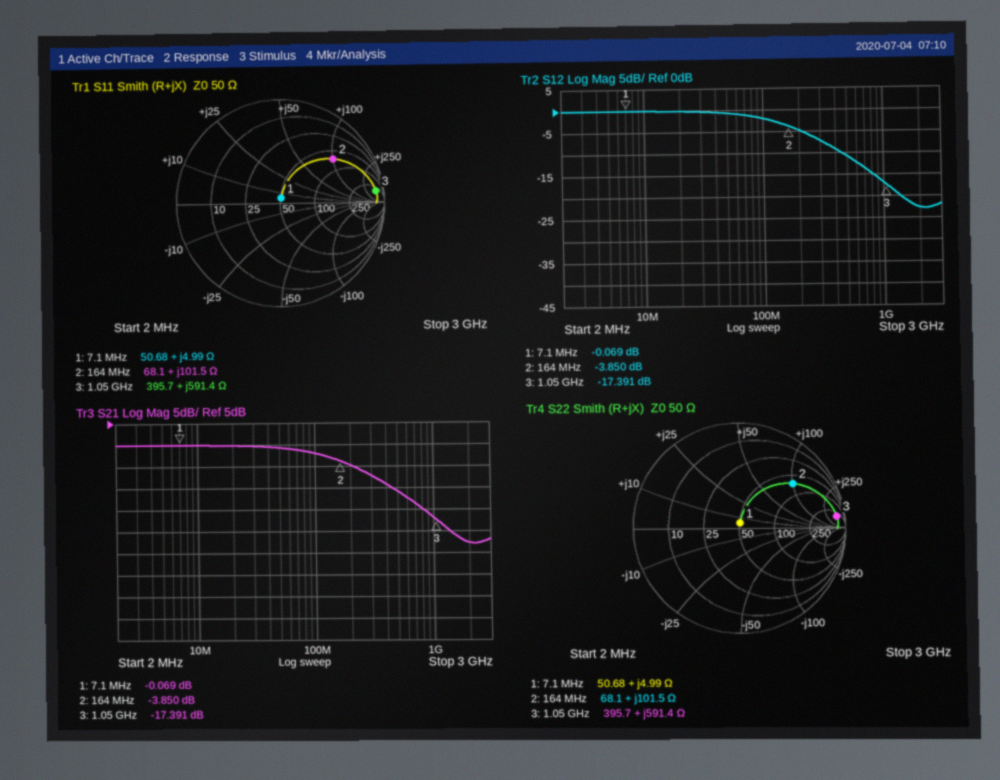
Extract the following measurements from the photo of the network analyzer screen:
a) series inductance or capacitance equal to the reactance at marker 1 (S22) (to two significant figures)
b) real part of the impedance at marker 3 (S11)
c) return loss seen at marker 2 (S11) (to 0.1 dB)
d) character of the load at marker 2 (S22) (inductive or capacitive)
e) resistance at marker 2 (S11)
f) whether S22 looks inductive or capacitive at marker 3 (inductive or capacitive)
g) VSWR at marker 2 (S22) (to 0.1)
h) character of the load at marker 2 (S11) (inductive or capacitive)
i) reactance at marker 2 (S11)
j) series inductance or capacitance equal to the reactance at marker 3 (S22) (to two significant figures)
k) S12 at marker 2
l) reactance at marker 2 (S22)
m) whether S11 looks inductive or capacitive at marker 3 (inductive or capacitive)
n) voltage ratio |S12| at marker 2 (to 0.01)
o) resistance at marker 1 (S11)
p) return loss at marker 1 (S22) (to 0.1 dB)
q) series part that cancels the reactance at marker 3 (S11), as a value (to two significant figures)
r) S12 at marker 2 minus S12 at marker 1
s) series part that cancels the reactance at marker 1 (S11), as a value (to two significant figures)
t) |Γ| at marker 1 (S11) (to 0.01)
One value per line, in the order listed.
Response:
110 nH
395.7 Ω
3.6 dB
inductive
68.1 Ω
inductive
4.9
inductive
+101.5 Ω
90 nH
-3.850 dB
+101.5 Ω
inductive
0.64
50.68 Ω
26.0 dB
260 fF
-3.781 dB
4.5 nF
0.05
